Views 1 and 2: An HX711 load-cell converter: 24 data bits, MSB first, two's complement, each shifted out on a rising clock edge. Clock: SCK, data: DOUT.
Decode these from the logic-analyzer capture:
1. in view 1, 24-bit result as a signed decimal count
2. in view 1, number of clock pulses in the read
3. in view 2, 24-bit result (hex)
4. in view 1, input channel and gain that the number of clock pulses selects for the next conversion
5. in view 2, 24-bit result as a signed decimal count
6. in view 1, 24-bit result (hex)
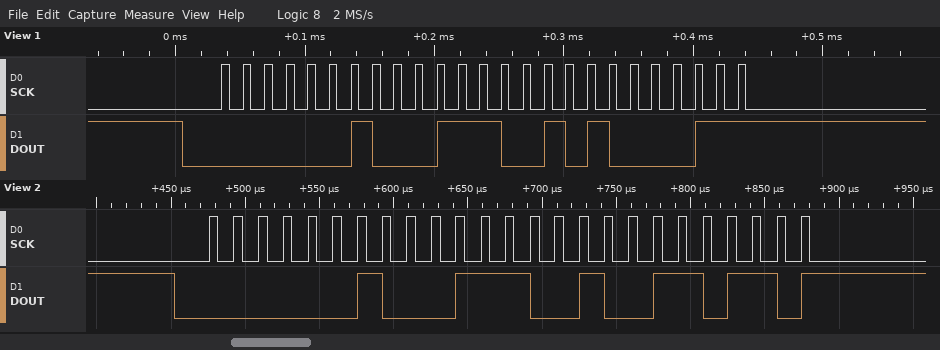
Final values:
145731
25
0x023936
channel A, gain 128
145718
0x023943
